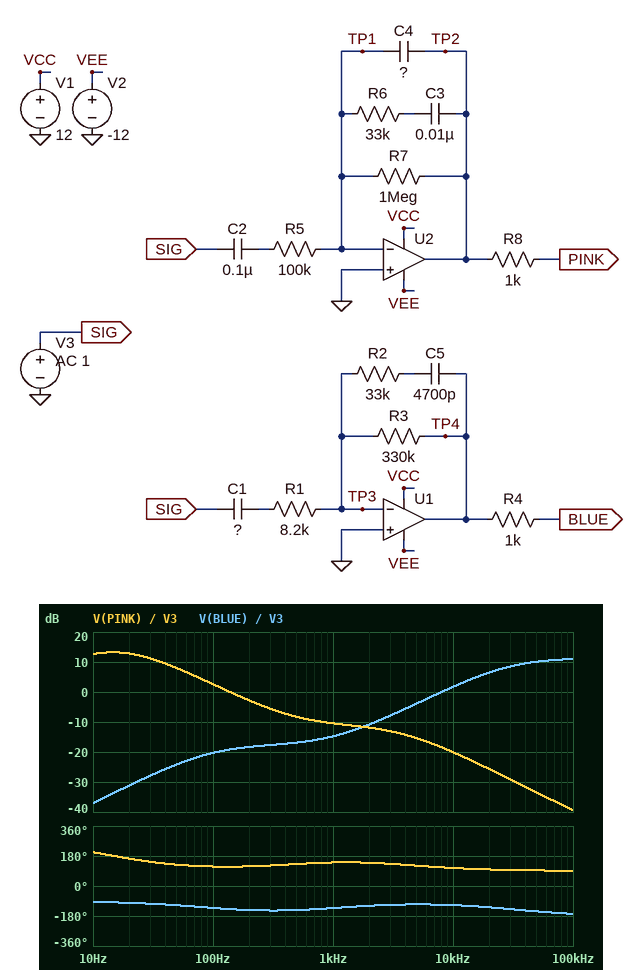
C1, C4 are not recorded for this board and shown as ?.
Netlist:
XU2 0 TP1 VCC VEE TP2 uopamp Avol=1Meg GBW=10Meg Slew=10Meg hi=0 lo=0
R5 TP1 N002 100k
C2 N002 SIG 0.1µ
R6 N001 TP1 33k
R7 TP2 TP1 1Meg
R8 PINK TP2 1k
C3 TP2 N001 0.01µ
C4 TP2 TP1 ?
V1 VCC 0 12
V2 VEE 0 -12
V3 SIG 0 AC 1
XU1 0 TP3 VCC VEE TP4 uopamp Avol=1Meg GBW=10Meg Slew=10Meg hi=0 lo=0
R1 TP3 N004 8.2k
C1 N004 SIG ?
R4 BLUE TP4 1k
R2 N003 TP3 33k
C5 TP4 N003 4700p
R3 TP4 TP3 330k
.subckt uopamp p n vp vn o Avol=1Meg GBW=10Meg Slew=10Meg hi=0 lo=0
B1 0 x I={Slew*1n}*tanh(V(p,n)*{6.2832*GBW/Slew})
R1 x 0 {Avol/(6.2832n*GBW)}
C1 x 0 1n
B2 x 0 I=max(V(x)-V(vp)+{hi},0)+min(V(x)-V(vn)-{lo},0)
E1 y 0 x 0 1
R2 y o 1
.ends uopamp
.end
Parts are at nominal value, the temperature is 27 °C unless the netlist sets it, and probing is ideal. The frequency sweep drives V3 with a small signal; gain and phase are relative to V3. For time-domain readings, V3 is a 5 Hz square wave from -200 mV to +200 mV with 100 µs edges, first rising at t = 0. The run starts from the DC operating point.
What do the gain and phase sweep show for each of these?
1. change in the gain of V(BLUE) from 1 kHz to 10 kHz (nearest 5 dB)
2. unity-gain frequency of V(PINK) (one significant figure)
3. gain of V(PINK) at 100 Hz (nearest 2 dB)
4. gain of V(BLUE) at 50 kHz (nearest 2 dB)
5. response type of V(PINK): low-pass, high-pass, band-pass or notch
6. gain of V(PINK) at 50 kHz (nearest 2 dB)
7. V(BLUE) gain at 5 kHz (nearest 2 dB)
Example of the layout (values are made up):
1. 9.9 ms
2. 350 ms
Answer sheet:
1. 15 dB
2. 100 Hz
3. 2 dB
4. 10 dB
5. low-pass
6. -34 dB
7. -4 dB
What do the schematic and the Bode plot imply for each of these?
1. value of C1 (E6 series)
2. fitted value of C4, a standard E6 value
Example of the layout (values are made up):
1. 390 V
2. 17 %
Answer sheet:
1. 680 pF
2. 1.5 nF
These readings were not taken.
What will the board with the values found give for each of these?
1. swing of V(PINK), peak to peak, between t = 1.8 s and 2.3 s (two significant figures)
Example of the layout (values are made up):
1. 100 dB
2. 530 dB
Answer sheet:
1. 2.7 V
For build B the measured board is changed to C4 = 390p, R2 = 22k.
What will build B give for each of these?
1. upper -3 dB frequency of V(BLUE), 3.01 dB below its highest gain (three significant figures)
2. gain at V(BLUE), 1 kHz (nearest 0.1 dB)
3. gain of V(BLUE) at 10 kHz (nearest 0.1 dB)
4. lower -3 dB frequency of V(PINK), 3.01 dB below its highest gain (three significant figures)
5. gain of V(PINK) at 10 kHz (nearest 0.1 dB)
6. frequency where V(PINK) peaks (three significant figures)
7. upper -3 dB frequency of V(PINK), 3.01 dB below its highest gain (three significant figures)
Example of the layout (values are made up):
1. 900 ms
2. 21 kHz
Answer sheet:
1. 2.88 MHz
2. -15.9 dB
3. -1.5 dB
4. 6.37 Hz
5. -12.2 dB
6. 15.4 Hz
7. 37.3 Hz
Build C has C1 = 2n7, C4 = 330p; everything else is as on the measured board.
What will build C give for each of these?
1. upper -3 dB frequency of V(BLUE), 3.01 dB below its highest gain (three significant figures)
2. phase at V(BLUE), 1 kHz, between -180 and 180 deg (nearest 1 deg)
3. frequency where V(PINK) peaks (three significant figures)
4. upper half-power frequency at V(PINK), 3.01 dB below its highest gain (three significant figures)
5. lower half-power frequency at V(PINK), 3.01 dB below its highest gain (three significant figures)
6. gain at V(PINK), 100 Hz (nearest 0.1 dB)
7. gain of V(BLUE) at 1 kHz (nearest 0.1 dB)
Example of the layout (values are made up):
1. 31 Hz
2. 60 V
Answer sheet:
1. 2.16 MHz
2. -138 deg
3. 15.4 Hz
4. 37.4 Hz
5. 6.39 Hz
6. 3.5 dB
7. -2.9 dB
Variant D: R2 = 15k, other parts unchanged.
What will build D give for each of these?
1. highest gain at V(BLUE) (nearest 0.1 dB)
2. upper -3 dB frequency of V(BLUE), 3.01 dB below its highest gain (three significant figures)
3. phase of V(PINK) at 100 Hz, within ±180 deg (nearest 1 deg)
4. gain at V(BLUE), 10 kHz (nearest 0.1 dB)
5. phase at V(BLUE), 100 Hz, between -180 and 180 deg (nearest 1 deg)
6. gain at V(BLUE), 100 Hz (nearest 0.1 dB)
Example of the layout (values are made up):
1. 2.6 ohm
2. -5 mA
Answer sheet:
1. 4.8 dB
2. 3.68 MHz
3. 117 deg
4. -4.5 dB
5. -133 deg
6. -20.1 dB
